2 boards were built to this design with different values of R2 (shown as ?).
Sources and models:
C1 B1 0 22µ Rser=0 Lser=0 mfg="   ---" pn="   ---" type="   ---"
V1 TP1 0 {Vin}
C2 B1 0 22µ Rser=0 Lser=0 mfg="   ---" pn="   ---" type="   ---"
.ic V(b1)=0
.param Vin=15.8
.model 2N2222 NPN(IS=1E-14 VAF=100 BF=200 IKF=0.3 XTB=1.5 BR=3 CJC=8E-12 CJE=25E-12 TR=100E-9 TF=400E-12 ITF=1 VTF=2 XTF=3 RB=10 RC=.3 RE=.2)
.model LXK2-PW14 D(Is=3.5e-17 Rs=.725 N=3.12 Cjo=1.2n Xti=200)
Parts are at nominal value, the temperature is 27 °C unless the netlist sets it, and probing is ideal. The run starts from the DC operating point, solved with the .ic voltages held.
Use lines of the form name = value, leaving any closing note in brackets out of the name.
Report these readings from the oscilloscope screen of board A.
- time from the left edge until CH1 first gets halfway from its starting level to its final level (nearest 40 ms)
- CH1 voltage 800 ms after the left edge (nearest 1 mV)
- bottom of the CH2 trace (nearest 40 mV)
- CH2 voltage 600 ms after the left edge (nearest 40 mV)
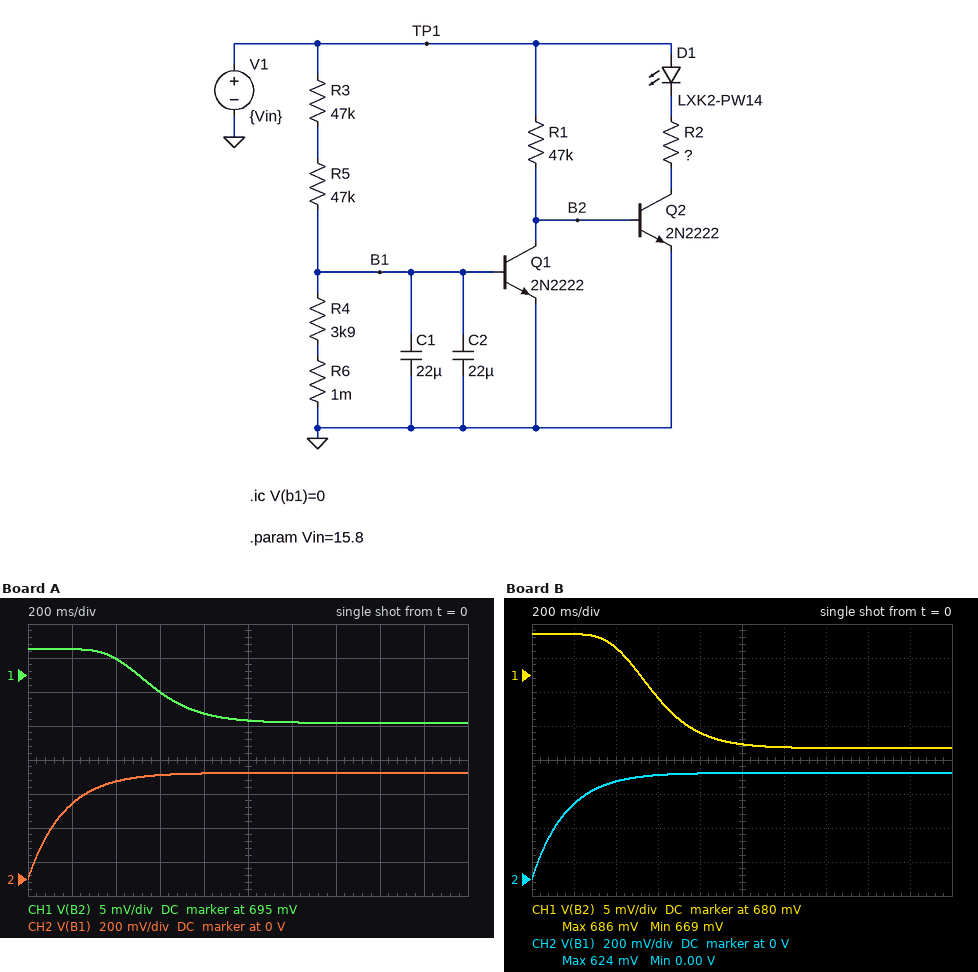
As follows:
time from the left edge until CH1 first gets halfway from its starting level to its final level = 560 ms
CH1 voltage 800 ms after the left edge = 689 mV
bottom of the CH2 trace = 0 V
CH2 voltage 600 ms after the left edge = 600 mV
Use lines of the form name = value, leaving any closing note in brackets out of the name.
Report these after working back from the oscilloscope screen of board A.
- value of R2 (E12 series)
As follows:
value of R2 = 3.9 kΩ
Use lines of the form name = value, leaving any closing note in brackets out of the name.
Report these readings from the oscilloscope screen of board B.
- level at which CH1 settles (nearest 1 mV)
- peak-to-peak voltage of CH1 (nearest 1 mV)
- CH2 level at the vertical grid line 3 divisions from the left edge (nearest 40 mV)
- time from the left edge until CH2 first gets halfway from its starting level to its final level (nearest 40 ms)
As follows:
level at which CH1 settles = 669 mV
peak-to-peak voltage of CH1 = 17 mV
CH2 level at the vertical grid line 3 divisions from the left edge = 600 mV
time from the left edge until CH2 first gets halfway from its starting level to its final level = 120 ms
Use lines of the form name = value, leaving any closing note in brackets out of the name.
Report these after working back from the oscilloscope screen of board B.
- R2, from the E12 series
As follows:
R2, from the E12 series = 8.2 kΩ
